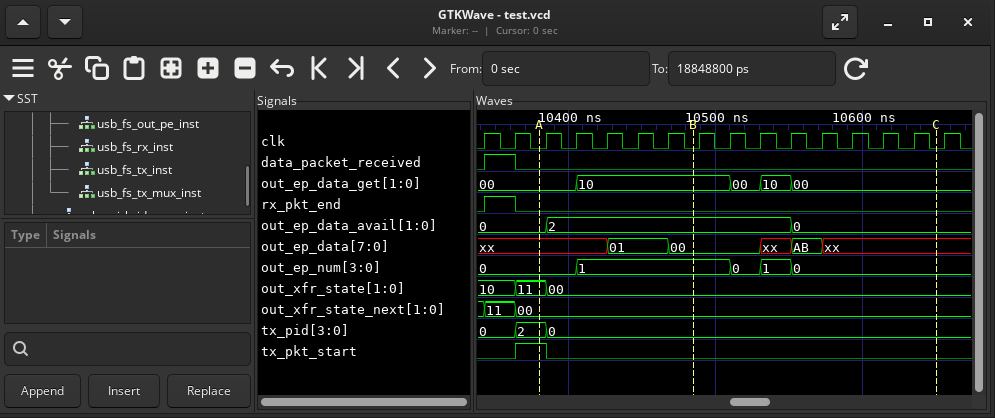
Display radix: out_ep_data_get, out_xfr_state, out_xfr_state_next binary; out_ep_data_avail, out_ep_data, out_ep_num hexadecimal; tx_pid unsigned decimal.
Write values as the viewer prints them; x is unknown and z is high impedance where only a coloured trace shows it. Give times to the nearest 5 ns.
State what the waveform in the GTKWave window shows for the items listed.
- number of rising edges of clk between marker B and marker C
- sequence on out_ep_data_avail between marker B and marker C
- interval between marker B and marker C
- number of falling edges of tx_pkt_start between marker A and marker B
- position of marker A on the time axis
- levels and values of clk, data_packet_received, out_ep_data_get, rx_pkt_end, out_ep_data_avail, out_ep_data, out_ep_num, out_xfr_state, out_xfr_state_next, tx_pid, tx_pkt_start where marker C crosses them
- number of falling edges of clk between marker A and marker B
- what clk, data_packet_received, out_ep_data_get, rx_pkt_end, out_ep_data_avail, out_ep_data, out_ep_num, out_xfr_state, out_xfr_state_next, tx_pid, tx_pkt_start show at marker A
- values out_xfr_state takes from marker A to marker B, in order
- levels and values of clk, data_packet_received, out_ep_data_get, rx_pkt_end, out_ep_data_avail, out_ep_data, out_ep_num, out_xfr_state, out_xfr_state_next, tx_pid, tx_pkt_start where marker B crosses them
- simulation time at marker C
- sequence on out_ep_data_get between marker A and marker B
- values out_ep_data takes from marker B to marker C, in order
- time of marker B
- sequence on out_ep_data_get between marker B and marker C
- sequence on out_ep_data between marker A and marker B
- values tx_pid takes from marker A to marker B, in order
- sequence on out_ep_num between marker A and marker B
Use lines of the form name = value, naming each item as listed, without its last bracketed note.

number of rising edges of clk between marker B and marker C = 8
sequence on out_ep_data_avail between marker B and marker C = 2, 0
interval between marker B and marker C = 165 ns
number of falling edges of tx_pkt_start between marker A and marker B = 1
position of marker A on the time axis = 10380 ns
levels and values of clk, data_packet_received, out_ep_data_get, rx_pkt_end, out_ep_data_avail, out_ep_data, out_ep_num, out_xfr_state, out_xfr_state_next, tx_pid, tx_pkt_start where marker C crosses them = clk=0, data_packet_received=0, out_ep_data_get=00, rx_pkt_end=0, out_ep_data_avail=0, out_ep_data=xx, out_ep_num=0, out_xfr_state=00, out_xfr_state_next=00, tx_pid=0, tx_pkt_start=0
number of falling edges of clk between marker A and marker B = 5
what clk, data_packet_received, out_ep_data_get, rx_pkt_end, out_ep_data_avail, out_ep_data, out_ep_num, out_xfr_state, out_xfr_state_next, tx_pid, tx_pkt_start show at marker A = clk=0, data_packet_received=0, out_ep_data_get=00, rx_pkt_end=0, out_ep_data_avail=0, out_ep_data=xx, out_ep_num=0, out_xfr_state=11, out_xfr_state_next=00, tx_pid=2, tx_pkt_start=1
values out_xfr_state takes from marker A to marker B, in order = 11, 00
levels and values of clk, data_packet_received, out_ep_data_get, rx_pkt_end, out_ep_data_avail, out_ep_data, out_ep_num, out_xfr_state, out_xfr_state_next, tx_pid, tx_pkt_start where marker B crosses them = clk=0, data_packet_received=0, out_ep_data_get=10, rx_pkt_end=0, out_ep_data_avail=2, out_ep_data=00, out_ep_num=1, out_xfr_state=00, out_xfr_state_next=00, tx_pid=0, tx_pkt_start=0
simulation time at marker C = 10650 ns
sequence on out_ep_data_get between marker A and marker B = 00, 10
values out_ep_data takes from marker B to marker C, in order = 00, xx, AB, xx
time of marker B = 10485 ns
sequence on out_ep_data_get between marker B and marker C = 10, 00, 10, 00
sequence on out_ep_data between marker A and marker B = xx, 01, 00
values tx_pid takes from marker A to marker B, in order = 2, 0
sequence on out_ep_num between marker A and marker B = 0, 1
